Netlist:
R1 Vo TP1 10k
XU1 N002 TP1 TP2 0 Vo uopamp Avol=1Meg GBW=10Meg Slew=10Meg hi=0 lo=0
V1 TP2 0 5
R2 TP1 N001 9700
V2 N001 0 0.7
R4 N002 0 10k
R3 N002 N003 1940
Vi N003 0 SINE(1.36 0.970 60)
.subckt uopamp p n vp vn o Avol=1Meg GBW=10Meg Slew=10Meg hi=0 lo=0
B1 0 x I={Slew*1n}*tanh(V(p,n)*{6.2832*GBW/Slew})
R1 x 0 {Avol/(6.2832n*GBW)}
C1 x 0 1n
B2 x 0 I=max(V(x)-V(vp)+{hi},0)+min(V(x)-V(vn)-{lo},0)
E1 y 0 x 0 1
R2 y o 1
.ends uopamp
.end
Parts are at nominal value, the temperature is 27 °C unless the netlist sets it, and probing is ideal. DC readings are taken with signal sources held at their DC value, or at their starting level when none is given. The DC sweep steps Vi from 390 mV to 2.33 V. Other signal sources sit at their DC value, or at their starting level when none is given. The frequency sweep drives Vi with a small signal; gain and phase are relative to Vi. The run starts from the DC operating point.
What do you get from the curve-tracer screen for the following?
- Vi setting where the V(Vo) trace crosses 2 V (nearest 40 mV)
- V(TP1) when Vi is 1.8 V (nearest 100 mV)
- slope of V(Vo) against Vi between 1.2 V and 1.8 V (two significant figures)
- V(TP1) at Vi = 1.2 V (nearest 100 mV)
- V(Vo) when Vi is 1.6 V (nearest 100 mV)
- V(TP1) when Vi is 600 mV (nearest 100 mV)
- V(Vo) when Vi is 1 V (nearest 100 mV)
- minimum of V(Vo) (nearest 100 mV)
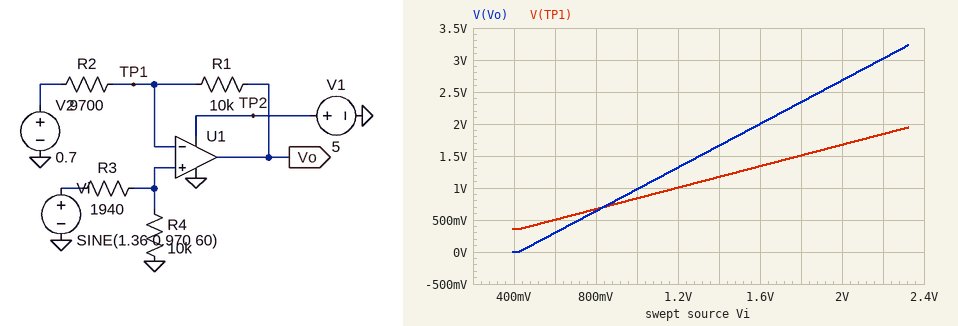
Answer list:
1.60 V
1.5 V
1.7 V/V
1.0 V
2.0 V
500 mV
1.0 V
0 V
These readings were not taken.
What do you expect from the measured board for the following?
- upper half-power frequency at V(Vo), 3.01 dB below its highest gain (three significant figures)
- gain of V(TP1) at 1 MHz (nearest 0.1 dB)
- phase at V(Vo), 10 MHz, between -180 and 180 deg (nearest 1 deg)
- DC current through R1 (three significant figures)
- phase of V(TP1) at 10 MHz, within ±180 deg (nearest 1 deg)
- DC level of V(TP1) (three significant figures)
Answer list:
4.92 MHz
-1.7 dB
-64 deg
45.3 µA
-64 deg
1.14 V
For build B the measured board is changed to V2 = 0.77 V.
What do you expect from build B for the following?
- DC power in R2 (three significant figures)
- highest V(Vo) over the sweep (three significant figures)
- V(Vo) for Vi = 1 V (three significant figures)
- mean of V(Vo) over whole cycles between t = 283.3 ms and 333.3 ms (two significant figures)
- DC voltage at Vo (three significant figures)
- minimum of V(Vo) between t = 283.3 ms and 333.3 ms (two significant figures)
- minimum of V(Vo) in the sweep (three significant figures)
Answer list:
14.0 µW
3.17 V
907 mV
1.5 V
1.52 V
-3.7 mV
-3.69 mV
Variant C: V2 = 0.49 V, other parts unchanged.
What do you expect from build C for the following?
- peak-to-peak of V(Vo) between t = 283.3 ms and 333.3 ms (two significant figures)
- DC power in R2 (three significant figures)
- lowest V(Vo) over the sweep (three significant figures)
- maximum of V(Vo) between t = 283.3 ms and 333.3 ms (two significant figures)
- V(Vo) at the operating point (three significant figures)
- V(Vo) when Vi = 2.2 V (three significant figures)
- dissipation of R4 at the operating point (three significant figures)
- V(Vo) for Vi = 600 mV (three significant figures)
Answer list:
3.3 V
43.4 µW
158 mV
3.5 V
1.81 V
3.24 V
130 µW
515 mV
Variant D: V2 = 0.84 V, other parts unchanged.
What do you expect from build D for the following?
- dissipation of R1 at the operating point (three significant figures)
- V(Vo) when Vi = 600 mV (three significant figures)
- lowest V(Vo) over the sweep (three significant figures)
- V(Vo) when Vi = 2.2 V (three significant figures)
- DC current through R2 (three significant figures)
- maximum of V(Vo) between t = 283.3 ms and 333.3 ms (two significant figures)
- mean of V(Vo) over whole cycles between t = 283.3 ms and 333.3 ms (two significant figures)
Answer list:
9.50 µW
155 mV
-5.40 mV
2.88 V
30.8 µA
3.1 V
1.5 V
